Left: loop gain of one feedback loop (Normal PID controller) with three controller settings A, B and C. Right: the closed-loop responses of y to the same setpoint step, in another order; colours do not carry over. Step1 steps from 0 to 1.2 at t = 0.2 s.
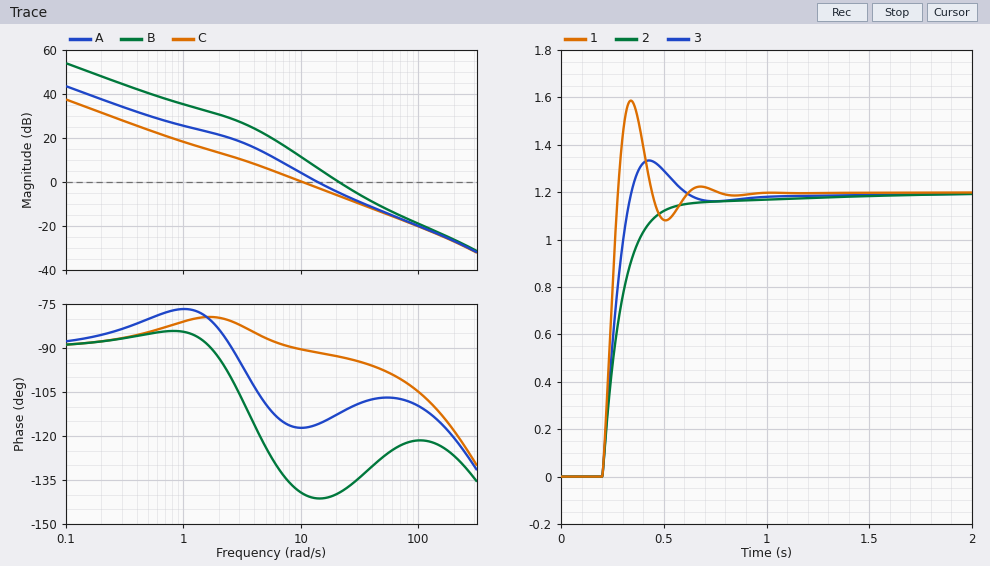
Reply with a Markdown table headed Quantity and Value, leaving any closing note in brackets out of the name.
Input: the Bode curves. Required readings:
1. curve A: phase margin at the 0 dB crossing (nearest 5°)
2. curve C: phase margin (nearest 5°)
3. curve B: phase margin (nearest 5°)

| Quantity | Value |
|---|---|
| curve A: phase margin at the 0 dB crossing | 65° |
| curve C: phase margin | 90° |
| curve B: phase margin | 40° |
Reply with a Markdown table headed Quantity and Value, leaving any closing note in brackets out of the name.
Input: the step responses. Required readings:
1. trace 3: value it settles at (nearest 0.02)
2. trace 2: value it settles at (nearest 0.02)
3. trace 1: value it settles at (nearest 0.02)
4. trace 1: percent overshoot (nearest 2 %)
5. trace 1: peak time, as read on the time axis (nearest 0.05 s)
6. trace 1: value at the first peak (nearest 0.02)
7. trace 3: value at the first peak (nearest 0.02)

| Quantity | Value |
|---|---|
| trace 3: value it settles at | 1.20 |
| trace 2: value it settles at | 1.20 |
| trace 1: value it settles at | 1.20 |
| trace 1: percent overshoot | 32 % |
| trace 1: peak time, as read on the time axis | 0.35 s |
| trace 1: value at the first peak | 1.58 |
| trace 3: value at the first peak | 1.34 |
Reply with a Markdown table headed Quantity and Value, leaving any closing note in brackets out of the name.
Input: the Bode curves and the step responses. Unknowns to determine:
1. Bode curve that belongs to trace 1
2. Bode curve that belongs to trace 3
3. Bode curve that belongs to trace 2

| Quantity | Value |
|---|---|
| Bode curve that belongs to trace 1 | B |
| Bode curve that belongs to trace 3 | A |
| Bode curve that belongs to trace 2 | C |
